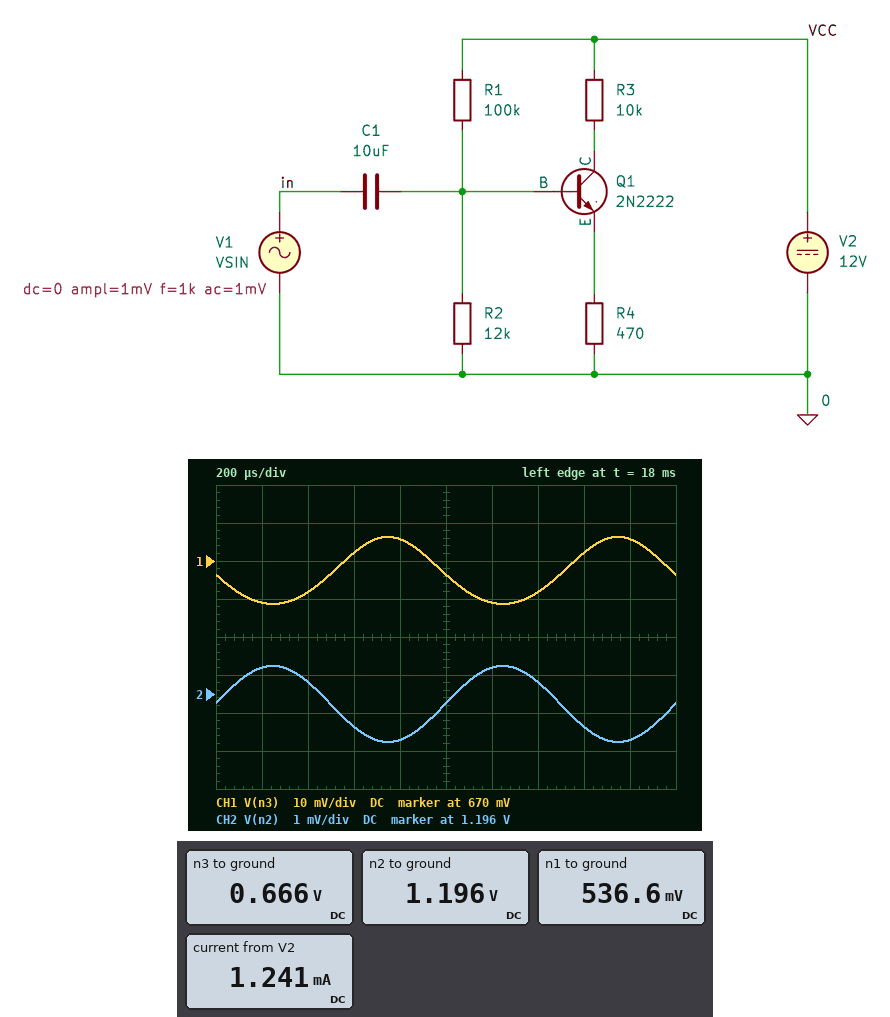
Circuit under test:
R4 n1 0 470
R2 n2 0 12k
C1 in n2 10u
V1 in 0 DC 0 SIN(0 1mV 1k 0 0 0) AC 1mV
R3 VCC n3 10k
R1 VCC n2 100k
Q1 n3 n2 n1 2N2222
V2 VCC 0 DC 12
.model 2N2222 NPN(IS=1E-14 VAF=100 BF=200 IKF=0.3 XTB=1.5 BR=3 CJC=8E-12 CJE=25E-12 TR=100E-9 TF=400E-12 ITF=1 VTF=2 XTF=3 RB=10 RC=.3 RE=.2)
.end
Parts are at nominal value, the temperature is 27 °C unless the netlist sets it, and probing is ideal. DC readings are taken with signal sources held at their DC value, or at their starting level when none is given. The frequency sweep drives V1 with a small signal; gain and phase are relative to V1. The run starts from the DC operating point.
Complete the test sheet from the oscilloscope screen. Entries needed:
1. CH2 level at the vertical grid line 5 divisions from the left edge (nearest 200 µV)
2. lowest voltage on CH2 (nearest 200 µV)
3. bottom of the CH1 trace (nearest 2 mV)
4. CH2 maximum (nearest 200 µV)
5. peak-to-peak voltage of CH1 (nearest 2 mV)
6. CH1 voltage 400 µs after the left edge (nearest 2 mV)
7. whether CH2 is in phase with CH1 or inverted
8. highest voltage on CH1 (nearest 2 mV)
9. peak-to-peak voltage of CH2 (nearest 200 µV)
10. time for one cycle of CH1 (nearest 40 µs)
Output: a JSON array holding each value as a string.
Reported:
["1.1958 V", "1.1948 V", "658 mV", "1.1968 V", "18 mV", "662 mV", "inverted", "676 mV", "2.0 mV", "1.00 ms"]
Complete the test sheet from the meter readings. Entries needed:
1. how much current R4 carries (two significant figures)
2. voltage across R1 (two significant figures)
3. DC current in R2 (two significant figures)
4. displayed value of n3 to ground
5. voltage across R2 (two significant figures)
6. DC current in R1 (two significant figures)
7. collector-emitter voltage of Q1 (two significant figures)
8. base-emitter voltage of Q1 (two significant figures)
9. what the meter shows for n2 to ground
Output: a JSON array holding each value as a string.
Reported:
["1.1 mA", "11 V", "100 µA", "0.666 V", "1.2 V", "110 µA", "130 mV", "660 mV", "1.196 V"]
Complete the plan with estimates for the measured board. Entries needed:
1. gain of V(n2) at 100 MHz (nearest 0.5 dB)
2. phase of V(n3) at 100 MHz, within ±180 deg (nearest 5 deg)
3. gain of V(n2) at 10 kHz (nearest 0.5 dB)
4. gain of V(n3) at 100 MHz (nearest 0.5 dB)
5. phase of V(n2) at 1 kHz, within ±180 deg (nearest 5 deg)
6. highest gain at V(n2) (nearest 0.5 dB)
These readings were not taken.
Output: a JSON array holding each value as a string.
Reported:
["0 dB", "5 deg", "0 dB", "0 dB", "0 deg", "0 dB"]
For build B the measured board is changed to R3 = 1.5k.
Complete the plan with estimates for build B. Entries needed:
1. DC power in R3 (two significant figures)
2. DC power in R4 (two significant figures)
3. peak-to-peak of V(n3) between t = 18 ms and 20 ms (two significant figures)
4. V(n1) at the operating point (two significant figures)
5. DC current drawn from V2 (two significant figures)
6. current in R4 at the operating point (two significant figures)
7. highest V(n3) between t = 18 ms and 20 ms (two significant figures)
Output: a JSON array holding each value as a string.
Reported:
["2.2 mW", "690 µW", "6.1 mV", "570 mV", "1.3 mA", "1.2 mA", "10 V"]
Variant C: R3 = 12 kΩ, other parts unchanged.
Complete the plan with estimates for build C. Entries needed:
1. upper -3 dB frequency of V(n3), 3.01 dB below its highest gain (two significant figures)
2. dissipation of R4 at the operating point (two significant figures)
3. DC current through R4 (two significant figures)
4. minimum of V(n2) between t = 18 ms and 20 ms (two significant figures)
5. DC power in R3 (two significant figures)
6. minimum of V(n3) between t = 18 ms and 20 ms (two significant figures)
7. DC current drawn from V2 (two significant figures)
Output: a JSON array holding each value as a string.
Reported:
["790 kHz", "440 µW", "970 µA", "1.1 V", "11 mW", "540 mV", "1.1 mA"]
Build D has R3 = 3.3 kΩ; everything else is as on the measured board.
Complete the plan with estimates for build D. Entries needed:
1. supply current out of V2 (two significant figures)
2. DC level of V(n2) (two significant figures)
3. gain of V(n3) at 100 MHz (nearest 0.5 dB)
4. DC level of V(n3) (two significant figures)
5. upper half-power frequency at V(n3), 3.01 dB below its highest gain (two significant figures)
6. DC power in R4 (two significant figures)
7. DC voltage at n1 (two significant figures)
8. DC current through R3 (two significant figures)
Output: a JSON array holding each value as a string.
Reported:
["1.3 mA", "1.2 V", "3.5 dB", "8.0 V", "13 MHz", "680 µW", "570 mV", "1.2 mA"]
